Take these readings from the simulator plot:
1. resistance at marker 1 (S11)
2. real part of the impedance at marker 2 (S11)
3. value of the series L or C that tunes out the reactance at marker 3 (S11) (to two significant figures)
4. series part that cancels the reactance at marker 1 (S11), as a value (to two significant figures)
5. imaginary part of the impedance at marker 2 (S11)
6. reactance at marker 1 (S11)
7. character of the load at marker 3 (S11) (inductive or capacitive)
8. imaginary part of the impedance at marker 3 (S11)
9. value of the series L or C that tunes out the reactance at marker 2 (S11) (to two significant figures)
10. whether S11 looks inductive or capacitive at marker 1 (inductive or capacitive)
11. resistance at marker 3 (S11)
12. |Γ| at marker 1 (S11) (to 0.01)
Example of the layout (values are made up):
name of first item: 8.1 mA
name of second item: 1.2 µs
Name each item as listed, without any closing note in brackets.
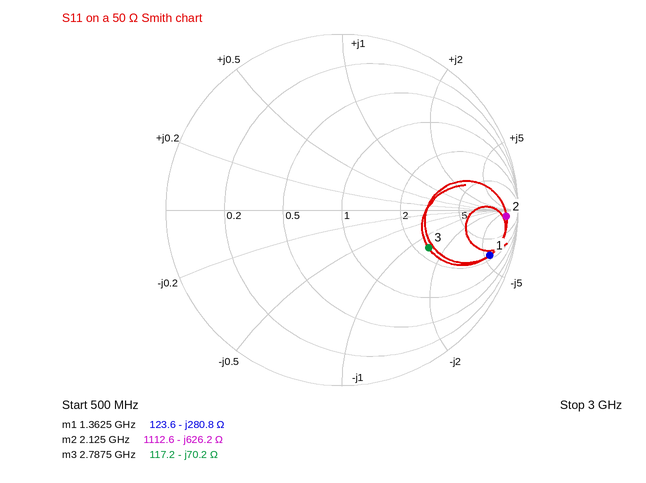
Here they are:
resistance at marker 1: 123.6 Ω
real part of the impedance at marker 2: 1112.6 Ω
value of the series L or C that tunes out the reactance at marker 3 (S11): 4.0 nH
series part that cancels the reactance at marker 1 (S11), as a value: 33 nH
imaginary part of the impedance at marker 2: -626.2 Ω
reactance at marker 1: -280.8 Ω
character of the load at marker 3 (S11): capacitive
imaginary part of the impedance at marker 3: -70.2 Ω
value of the series L or C that tunes out the reactance at marker 2 (S11): 47 nH
whether S11 looks inductive or capacitive at marker 1: capacitive
resistance at marker 3: 117.2 Ω
|Γ| at marker 1 (S11): 0.88
